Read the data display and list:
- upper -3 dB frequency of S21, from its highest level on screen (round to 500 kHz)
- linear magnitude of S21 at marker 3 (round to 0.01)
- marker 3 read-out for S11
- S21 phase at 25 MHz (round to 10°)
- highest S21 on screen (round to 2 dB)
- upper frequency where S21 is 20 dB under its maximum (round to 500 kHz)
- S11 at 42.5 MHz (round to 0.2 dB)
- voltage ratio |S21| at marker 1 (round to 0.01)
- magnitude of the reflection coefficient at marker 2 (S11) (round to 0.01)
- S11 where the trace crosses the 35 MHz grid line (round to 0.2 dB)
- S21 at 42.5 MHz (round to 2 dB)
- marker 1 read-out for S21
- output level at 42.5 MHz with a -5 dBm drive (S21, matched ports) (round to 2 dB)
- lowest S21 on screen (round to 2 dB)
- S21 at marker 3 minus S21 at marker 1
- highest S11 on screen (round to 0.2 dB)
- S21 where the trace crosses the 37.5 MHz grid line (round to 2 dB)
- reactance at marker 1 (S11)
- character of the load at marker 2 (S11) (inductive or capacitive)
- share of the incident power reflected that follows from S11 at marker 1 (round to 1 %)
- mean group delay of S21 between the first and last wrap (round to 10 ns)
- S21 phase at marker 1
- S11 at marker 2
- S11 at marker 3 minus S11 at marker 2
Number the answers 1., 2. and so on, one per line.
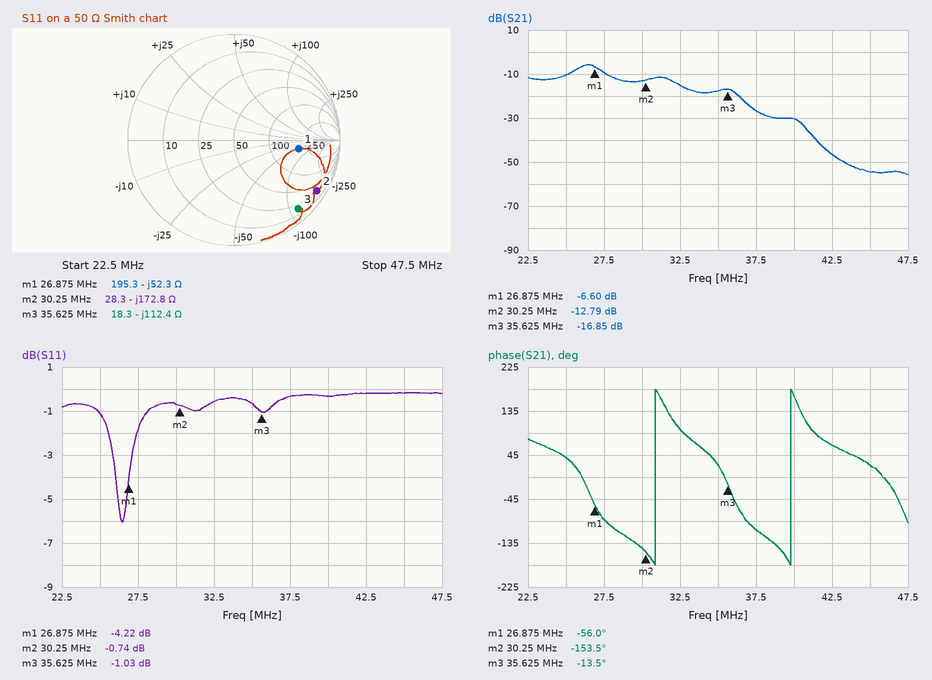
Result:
1. 27.5 MHz
2. 0.14
3. -1.03 dB
4. 40°
5. -6 dB
6. 37.5 MHz
7. -0.2 dB
8. 0.47
9. 0.92
10. -0.6 dB
11. -46 dB
12. -6.60 dB
13. -52 dBm
14. -56 dB
15. -10.25 dB
16. -0.2 dB
17. -26 dB
18. -52.3 Ω
19. capacitive
20. 38 %
21. 110 ns
22. -56.0°
23. -0.74 dB
24. -0.29 dB
